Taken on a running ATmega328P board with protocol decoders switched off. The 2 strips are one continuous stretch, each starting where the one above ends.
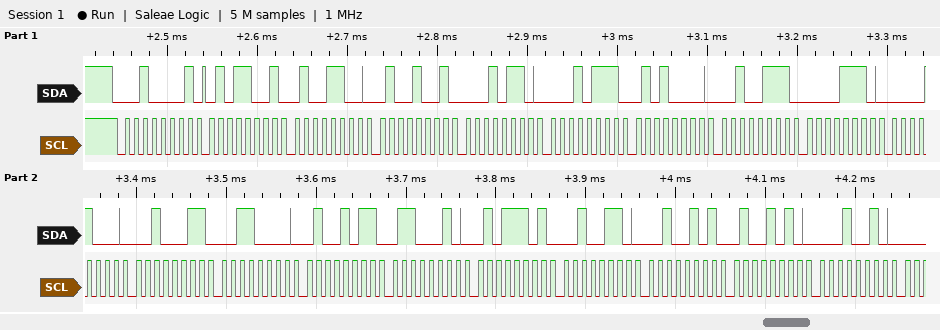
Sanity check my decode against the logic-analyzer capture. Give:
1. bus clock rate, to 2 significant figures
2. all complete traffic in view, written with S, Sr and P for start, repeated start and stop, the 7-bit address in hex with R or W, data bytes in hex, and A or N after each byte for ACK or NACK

100 kHz
S 10R A 59 A 4C A 49 A 16 A 17 A 50 A 27 A 0E A 08 A 23 A 30 A 4B A 62 A 5D A 26 A 25 A 4A A 12 A
